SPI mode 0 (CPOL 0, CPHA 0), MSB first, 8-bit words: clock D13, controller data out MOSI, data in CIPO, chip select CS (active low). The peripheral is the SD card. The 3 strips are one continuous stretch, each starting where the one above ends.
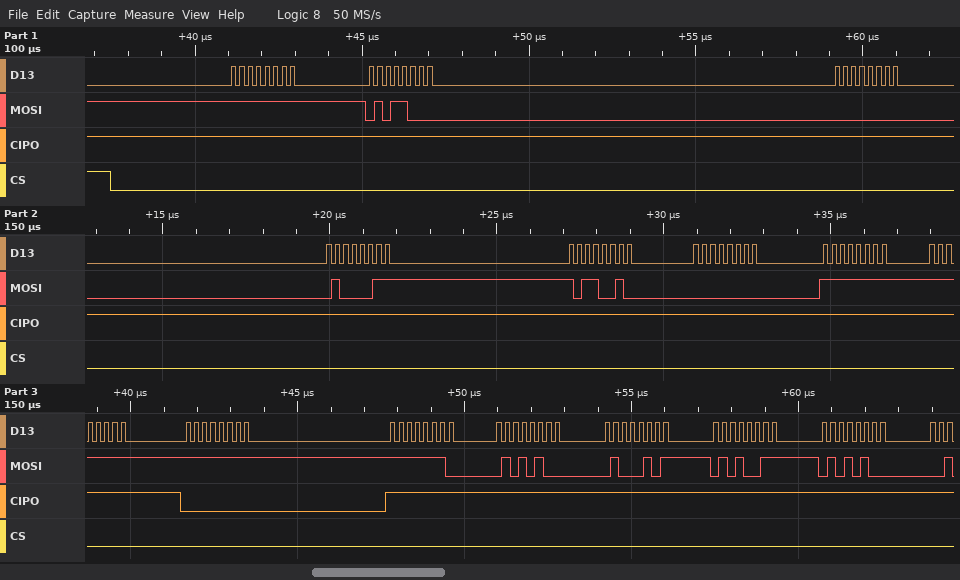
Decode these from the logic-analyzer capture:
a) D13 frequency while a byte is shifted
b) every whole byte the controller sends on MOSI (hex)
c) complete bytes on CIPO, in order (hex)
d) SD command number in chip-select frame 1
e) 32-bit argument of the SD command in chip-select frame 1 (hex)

4 MHz
FF 58 00 43 B2 00 FF FF FF FE 54 45 53 54
FF FF FF FF FF FF FF FF 00 FF FF FF FF FF
CMD24
0x0043B200
